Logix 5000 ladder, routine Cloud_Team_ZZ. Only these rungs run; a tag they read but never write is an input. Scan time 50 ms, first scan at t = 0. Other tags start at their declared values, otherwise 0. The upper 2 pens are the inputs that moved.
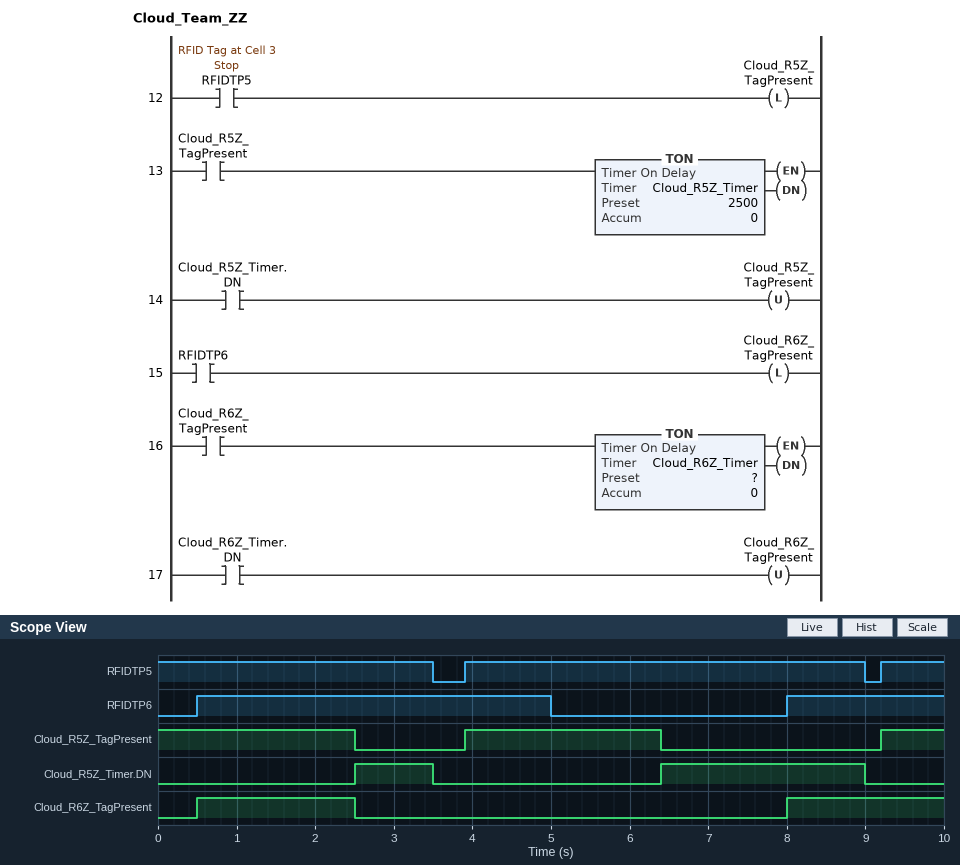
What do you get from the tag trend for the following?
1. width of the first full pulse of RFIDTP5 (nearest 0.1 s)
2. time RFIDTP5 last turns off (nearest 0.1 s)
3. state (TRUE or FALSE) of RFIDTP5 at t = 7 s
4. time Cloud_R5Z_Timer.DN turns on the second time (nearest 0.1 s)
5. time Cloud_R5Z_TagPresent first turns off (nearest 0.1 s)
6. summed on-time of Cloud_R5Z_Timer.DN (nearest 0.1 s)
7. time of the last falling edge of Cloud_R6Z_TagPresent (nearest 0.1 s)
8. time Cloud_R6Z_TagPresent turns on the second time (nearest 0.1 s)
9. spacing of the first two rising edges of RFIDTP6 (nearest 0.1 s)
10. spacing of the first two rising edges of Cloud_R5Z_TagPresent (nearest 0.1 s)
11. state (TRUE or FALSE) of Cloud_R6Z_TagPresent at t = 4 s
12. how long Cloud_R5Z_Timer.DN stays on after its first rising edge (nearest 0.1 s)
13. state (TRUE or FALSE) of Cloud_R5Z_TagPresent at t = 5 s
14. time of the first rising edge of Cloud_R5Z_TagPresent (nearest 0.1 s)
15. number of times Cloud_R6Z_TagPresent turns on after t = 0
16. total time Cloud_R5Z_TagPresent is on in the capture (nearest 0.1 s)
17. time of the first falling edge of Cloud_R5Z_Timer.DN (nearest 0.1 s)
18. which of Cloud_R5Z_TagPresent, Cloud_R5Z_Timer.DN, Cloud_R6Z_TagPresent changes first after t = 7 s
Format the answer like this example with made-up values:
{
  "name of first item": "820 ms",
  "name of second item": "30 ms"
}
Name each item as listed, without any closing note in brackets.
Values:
{
  "width of the first full pulse of RFIDTP5": "5.1 s",
  "time RFIDTP5 last turns off": "9.0 s",
  "state (TRUE or FALSE) of RFIDTP5 at t = 7 s": "TRUE",
  "time Cloud_R5Z_Timer.DN turns on the second time": "6.4 s",
  "time Cloud_R5Z_TagPresent first turns off": "2.5 s",
  "summed on-time of Cloud_R5Z_Timer.DN": "3.6 s",
  "time of the last falling edge of Cloud_R6Z_TagPresent": "2.5 s",
  "time Cloud_R6Z_TagPresent turns on the second time": "8.0 s",
  "spacing of the first two rising edges of RFIDTP6": "7.5 s",
  "spacing of the first two rising edges of Cloud_R5Z_TagPresent": "5.3 s",
  "state (TRUE or FALSE) of Cloud_R6Z_TagPresent at t = 4 s": "FALSE",
  "how long Cloud_R5Z_Timer.DN stays on after its first rising edge": "1.0 s",
  "state (TRUE or FALSE) of Cloud_R5Z_TagPresent at t = 5 s": "TRUE",
  "time of the first rising edge of Cloud_R5Z_TagPresent": "3.9 s",
  "number of times Cloud_R6Z_TagPresent turns on after t = 0": "2",
  "total time Cloud_R5Z_TagPresent is on in the capture": "5.8 s",
  "time of the first falling edge of Cloud_R5Z_Timer.DN": "3.5 s",
  "which of Cloud_R5Z_TagPresent, Cloud_R5Z_Timer.DN, Cloud_R6Z_TagPresent changes first after t = 7 s": "Cloud_R6Z_TagPresent"
}
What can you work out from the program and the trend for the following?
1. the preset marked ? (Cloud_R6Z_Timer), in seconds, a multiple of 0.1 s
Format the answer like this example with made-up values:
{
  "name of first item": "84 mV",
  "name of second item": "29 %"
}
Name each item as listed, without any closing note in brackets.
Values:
{
  "the preset marked ? (Cloud_R6Z_Timer), in seconds, a multiple of 0.1 s": "2.0 s"
}
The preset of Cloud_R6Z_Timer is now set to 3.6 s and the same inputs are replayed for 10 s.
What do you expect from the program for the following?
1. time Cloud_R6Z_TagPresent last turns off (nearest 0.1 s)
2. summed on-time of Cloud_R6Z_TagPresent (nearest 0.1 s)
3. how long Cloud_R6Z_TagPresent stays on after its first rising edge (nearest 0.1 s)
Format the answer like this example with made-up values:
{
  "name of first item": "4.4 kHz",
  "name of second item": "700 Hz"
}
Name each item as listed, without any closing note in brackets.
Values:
{
  "time Cloud_R6Z_TagPresent last turns off": "4.1 s",
  "summed on-time of Cloud_R6Z_TagPresent": "5.6 s",
  "how long Cloud_R6Z_TagPresent stays on after its first rising edge": "3.6 s"
}
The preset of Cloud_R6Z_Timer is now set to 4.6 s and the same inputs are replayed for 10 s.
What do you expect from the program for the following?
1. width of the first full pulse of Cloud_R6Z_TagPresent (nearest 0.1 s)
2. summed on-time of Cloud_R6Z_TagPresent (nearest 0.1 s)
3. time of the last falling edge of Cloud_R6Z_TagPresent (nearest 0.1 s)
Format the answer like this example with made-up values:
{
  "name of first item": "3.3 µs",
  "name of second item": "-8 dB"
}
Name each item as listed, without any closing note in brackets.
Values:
{
  "width of the first full pulse of Cloud_R6Z_TagPresent": "4.6 s",
  "summed on-time of Cloud_R6Z_TagPresent": "6.6 s",
  "time of the last falling edge of Cloud_R6Z_TagPresent": "5.1 s"
}
